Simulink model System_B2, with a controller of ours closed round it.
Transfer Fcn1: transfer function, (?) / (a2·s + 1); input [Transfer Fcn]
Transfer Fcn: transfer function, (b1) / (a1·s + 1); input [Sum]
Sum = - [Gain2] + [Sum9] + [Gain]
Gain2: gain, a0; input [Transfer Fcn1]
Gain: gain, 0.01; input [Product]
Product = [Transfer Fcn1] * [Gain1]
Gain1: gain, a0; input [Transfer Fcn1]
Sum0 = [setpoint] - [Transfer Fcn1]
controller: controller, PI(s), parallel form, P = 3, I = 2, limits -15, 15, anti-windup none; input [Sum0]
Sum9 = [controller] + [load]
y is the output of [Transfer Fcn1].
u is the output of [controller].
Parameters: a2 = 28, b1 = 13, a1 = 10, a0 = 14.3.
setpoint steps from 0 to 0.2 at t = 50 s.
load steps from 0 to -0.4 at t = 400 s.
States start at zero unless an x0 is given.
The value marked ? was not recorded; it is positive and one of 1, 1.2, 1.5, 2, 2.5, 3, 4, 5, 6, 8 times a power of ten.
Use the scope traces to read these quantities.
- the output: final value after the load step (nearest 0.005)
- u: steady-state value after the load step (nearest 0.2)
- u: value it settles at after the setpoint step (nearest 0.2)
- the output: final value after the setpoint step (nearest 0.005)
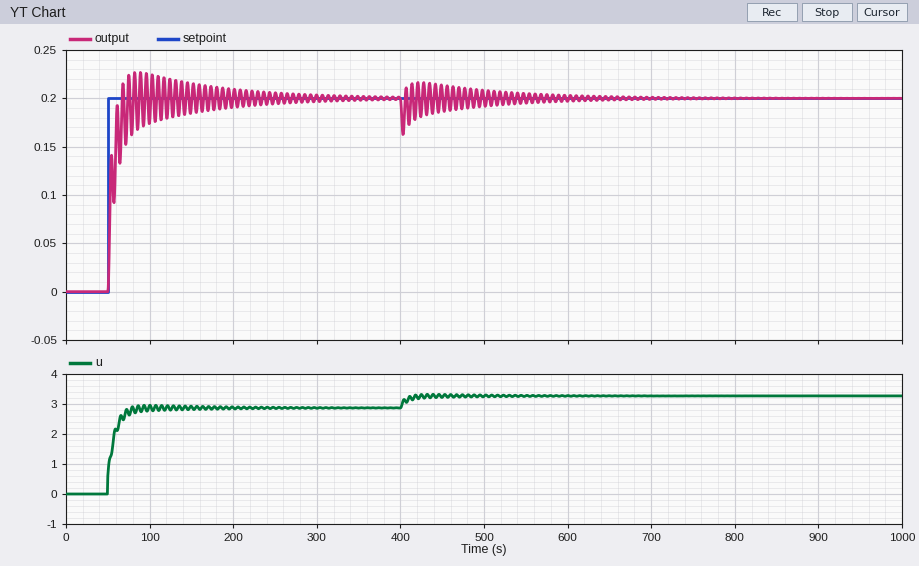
0.200
3.2
2.8
0.200
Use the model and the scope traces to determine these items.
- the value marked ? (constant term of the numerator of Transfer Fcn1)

1
